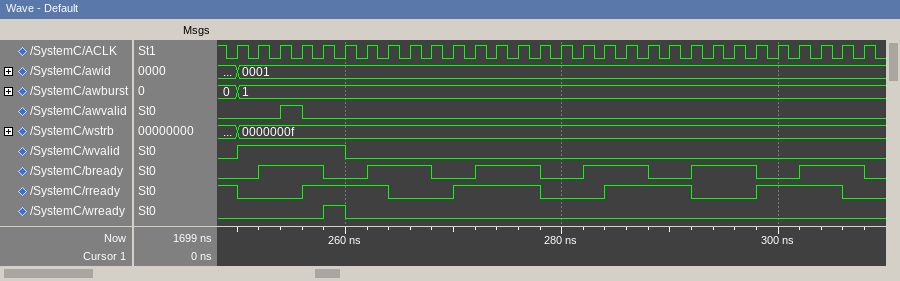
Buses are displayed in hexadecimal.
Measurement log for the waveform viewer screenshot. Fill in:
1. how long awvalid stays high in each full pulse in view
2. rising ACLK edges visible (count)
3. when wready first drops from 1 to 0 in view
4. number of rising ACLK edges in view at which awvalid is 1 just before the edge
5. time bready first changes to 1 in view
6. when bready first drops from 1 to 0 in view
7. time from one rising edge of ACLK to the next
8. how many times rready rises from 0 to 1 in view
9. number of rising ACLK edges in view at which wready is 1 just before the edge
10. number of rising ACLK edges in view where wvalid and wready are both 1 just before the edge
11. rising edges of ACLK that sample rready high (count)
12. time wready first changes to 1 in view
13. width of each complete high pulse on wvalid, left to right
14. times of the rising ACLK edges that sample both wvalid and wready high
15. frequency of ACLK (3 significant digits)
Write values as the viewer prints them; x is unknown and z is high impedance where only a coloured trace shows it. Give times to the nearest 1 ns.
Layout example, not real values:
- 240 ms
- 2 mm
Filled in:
- 2 ns
- 30
- 260 ns
- 1
- 252 ns
- 258 ns
- 2 ns
- 4
- 1
- 1
- 17
- 258 ns
- 10 ns
- 260 ns
- 500 MHz
